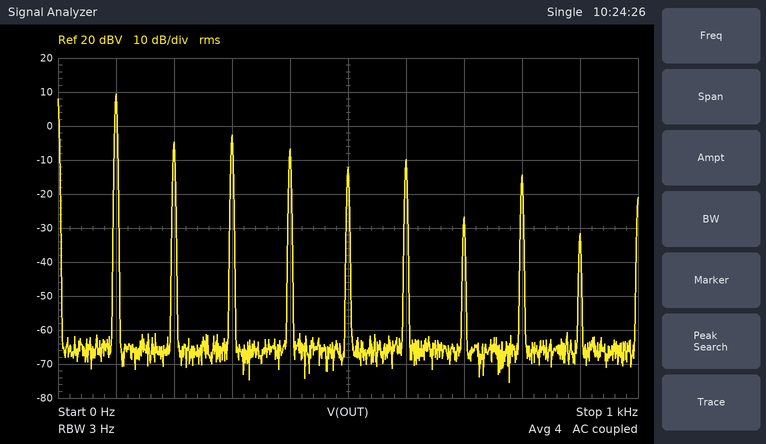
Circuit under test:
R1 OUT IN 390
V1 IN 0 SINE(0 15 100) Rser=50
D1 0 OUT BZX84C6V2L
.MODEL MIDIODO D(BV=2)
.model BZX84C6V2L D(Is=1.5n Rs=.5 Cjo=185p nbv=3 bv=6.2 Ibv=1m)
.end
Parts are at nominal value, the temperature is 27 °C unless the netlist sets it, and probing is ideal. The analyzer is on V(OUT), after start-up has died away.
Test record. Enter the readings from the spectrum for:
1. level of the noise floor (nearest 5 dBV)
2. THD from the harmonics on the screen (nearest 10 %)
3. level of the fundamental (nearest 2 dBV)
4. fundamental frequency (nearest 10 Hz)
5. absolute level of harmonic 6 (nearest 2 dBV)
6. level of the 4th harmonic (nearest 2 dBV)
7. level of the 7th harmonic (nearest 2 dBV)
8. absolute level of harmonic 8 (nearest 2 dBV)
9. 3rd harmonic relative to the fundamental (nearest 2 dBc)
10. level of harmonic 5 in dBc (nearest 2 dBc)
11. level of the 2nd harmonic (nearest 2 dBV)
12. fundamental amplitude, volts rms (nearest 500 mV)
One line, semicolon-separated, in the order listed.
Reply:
-65 dBV; 40 %; 10 dBV; 100 Hz; -10 dBV; -6 dBV; -26 dBV; -14 dBV; -12 dBc; -22 dBc; -4 dBV; 3.0 V
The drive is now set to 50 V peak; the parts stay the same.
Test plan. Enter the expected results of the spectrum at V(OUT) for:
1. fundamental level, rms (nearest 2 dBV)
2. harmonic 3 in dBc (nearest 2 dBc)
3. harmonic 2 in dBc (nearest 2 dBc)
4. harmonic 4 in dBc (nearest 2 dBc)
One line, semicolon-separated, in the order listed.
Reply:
10 dBV; -10 dBc; -24 dBc; -24 dBc
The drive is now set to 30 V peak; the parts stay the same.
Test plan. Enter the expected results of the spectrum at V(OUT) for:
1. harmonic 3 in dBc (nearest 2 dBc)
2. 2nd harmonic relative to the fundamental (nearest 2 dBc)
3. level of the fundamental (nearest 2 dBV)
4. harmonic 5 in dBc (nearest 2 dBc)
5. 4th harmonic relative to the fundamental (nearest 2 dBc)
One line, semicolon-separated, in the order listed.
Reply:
-10 dBc; -20 dBc; 10 dBV; -16 dBc; -20 dBc
